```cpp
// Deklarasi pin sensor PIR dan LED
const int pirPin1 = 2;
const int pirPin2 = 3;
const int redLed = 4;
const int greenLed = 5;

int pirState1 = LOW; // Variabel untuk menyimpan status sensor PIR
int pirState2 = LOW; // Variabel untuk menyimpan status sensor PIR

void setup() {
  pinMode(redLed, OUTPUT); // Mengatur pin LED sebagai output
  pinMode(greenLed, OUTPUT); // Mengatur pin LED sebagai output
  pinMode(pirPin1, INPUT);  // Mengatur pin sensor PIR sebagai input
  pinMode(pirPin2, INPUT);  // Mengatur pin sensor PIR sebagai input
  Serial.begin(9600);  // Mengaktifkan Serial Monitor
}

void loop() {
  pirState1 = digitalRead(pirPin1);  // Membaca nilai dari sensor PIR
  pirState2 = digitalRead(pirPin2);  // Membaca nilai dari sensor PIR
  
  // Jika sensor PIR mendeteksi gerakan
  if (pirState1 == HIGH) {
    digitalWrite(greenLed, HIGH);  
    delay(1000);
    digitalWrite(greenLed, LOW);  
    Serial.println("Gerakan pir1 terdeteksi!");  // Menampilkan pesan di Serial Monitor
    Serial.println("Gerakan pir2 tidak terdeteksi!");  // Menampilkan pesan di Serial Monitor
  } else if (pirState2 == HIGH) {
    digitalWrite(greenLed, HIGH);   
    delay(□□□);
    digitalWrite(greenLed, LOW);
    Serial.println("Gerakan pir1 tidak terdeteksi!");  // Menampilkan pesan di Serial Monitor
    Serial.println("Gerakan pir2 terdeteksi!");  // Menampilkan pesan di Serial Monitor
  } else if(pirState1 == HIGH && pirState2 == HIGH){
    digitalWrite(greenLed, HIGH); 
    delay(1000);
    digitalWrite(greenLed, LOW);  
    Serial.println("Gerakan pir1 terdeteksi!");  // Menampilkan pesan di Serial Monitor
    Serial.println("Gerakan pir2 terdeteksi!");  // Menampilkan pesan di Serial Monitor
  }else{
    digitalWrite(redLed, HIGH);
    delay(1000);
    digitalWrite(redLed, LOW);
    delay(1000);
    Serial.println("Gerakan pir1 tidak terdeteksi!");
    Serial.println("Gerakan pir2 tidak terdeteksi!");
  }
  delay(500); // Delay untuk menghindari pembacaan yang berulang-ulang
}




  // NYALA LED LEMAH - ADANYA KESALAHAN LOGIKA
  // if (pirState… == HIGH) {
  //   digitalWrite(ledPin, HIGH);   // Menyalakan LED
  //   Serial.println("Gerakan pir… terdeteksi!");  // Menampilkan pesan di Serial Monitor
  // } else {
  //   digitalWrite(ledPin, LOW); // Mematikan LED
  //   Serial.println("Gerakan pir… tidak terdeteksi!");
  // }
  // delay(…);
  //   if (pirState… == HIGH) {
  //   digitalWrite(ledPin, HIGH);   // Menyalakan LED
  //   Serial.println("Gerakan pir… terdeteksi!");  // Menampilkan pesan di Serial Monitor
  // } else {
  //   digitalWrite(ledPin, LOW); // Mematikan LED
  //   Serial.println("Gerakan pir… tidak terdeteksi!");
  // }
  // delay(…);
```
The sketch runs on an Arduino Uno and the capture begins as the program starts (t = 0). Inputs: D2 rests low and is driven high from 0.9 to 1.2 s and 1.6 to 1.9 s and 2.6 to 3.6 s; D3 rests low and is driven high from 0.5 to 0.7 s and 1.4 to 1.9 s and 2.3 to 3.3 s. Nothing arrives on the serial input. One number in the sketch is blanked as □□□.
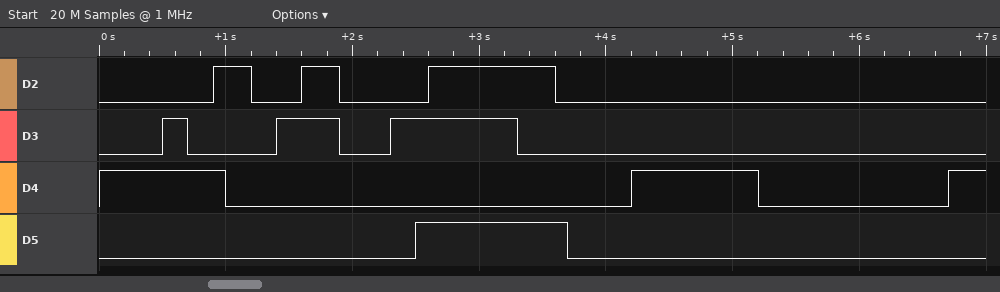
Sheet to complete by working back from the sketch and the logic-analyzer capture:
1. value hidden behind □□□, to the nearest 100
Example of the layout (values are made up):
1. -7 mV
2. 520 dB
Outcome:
1. 1200
